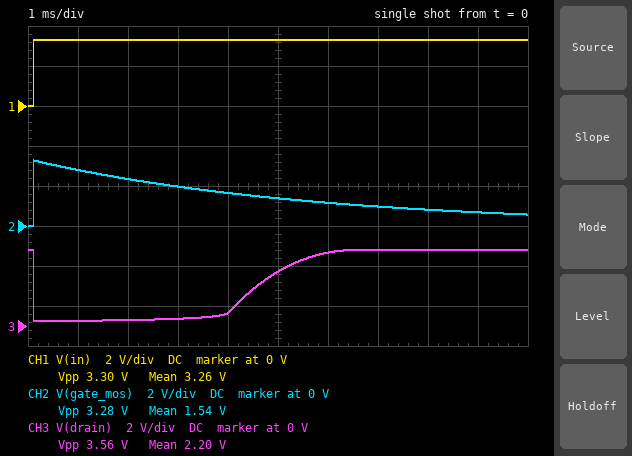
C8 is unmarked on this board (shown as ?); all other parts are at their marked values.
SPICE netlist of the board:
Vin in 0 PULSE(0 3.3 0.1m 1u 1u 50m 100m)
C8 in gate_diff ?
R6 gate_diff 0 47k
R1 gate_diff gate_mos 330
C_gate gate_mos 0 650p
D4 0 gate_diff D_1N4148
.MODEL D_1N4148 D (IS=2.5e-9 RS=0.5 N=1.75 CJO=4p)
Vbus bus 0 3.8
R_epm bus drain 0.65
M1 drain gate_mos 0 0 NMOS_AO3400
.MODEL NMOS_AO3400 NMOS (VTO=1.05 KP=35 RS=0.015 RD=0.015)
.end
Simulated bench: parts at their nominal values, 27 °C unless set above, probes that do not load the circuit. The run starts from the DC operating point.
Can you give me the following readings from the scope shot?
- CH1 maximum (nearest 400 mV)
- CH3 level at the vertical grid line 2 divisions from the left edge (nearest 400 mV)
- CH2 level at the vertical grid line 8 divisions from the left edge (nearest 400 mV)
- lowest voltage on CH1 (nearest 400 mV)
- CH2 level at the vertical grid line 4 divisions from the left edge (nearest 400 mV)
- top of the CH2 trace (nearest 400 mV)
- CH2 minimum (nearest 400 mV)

3.2 V
400 mV
800 mV
0 V
1.6 V
3.2 V
0 V
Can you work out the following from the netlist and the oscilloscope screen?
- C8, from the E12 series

120 nF
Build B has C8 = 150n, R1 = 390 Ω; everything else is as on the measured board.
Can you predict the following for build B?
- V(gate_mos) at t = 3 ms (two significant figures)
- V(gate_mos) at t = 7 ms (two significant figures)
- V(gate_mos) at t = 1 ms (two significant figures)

2.2 V
1.2 V
2.9 V
